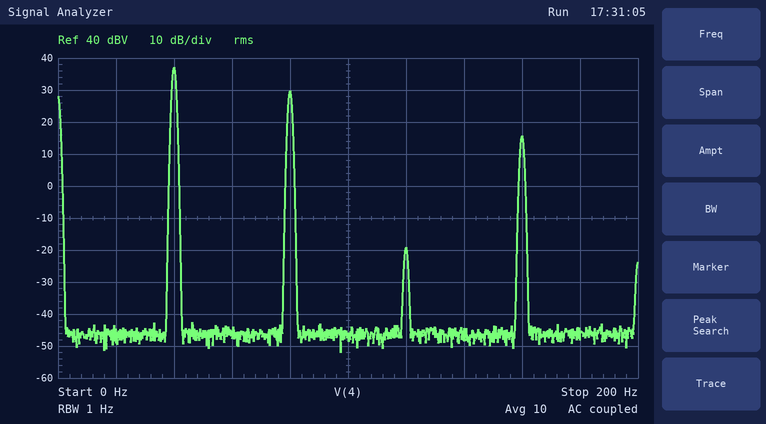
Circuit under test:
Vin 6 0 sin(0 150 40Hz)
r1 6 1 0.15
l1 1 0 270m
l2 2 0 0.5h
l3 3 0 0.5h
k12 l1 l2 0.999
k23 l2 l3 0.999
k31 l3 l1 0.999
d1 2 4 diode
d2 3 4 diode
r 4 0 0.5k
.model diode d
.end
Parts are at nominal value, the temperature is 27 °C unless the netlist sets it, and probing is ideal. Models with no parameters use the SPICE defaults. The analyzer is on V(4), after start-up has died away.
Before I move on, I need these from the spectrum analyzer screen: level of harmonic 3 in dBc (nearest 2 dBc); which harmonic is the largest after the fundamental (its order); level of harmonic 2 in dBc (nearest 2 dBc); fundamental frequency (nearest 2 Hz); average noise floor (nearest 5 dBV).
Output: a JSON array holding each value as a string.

["-56 dBc", "2", "-8 dBc", "40 Hz", "-45 dBV"]
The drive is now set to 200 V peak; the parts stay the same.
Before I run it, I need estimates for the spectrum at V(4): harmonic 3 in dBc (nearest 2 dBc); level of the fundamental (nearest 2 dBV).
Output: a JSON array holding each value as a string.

["-58 dBc", "40 dBV"]
